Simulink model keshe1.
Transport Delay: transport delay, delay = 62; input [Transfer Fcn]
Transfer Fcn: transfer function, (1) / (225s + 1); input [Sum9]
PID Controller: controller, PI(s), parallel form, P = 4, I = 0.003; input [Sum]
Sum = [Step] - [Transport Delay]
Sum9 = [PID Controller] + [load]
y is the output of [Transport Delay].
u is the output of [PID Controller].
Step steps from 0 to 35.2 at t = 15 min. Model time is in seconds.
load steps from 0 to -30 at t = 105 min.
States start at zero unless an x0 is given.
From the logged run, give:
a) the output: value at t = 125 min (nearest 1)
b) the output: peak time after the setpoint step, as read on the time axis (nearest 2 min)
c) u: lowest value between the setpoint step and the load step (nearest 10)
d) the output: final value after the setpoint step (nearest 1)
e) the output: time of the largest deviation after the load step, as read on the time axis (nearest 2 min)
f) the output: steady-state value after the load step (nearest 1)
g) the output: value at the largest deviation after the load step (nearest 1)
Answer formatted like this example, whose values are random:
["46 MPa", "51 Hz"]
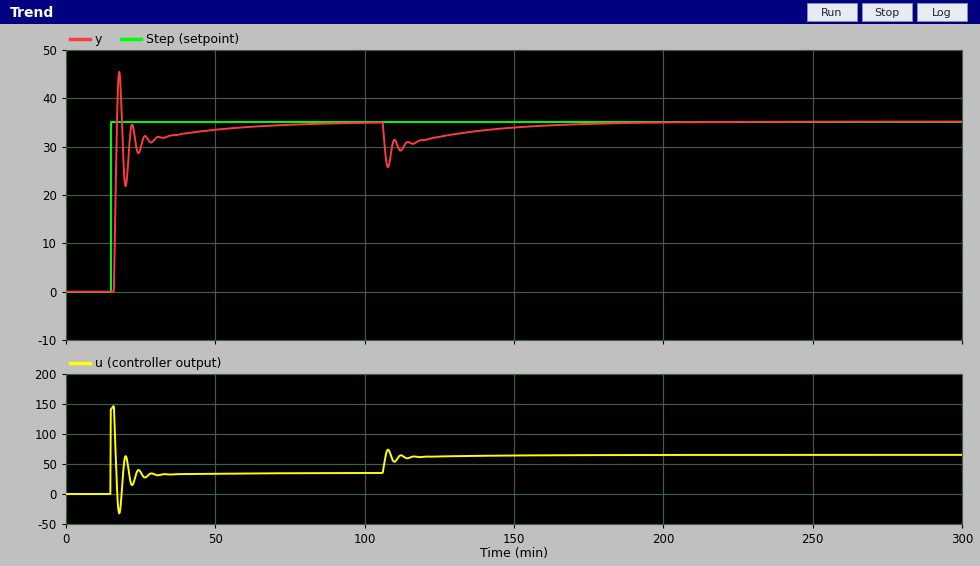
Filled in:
["32", "18 min", "-30", "35", "108 min", "35", "26"]
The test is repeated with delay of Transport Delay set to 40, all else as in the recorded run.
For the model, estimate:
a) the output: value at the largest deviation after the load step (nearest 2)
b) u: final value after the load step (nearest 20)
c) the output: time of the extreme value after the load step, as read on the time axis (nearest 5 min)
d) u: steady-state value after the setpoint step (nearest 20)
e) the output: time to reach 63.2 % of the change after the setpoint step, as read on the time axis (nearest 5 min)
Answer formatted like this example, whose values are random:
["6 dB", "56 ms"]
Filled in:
["28", "60", "105 min", "40", "15 min"]
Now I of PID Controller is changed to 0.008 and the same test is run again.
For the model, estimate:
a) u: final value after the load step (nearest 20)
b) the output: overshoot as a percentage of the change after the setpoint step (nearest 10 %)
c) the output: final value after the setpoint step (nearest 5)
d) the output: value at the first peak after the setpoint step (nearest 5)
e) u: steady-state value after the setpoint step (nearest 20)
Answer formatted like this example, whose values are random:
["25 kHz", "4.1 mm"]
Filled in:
["60", "40 %", "35", "50", "40"]
